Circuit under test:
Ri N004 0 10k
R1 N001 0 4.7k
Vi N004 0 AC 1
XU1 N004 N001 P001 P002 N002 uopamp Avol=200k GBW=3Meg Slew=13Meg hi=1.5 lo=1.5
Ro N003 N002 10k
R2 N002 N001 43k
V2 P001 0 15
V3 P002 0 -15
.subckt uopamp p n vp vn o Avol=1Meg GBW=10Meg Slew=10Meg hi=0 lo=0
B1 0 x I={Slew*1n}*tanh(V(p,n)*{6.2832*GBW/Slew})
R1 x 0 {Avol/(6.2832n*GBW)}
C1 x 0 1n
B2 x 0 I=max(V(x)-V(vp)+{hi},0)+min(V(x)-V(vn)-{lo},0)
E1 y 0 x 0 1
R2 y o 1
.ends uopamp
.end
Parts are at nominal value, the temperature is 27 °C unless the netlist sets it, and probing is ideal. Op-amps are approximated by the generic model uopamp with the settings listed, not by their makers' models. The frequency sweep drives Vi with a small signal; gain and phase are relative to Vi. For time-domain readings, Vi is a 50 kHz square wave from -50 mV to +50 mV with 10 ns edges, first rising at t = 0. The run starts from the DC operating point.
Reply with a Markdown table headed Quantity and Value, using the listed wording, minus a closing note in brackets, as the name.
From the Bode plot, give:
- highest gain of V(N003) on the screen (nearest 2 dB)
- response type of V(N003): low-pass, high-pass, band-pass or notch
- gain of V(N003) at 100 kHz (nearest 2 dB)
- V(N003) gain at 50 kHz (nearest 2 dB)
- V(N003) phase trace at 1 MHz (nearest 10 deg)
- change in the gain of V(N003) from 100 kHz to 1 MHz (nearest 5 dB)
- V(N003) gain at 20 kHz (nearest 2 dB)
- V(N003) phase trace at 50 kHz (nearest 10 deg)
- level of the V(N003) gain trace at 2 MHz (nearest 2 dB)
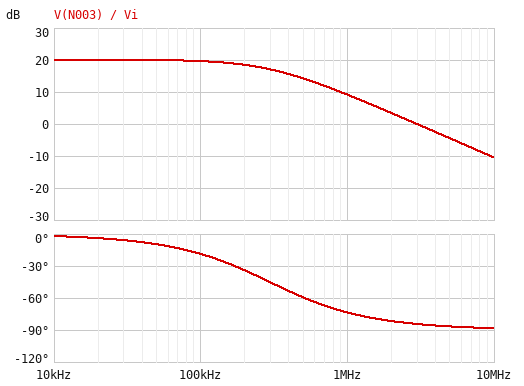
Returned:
| Quantity | Value |
|---|---|
| highest gain of V(N003) on the screen | 20 dB |
| response type of V(N003): low-pass, high-pass, band-pass or notch | low-pass |
| gain of V(N003) at 100 kHz | 20 dB |
| V(N003) gain at 50 kHz | 20 dB |
| V(N003) phase trace at 1 MHz | -70 deg |
| change in the gain of V(N003) from 100 kHz to 1 MHz | -10 dB |
| V(N003) gain at 20 kHz | 20 dB |
| V(N003) phase trace at 50 kHz | -10 deg |
| level of the V(N003) gain trace at 2 MHz | 4 dB |
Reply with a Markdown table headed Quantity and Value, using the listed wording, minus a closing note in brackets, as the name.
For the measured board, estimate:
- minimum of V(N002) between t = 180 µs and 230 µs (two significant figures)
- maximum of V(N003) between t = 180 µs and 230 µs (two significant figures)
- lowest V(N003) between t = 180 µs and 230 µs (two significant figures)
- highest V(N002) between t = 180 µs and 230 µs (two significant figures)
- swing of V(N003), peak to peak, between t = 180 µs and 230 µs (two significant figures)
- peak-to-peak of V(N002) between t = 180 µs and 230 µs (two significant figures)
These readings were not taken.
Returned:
| Quantity | Value |
|---|---|
| minimum of V(N002) between t = 180 µs and 230 µs | -510 mV |
| maximum of V(N003) between t = 180 µs and 230 µs | 510 mV |
| lowest V(N003) between t = 180 µs and 230 µs | -510 mV |
| highest V(N002) between t = 180 µs and 230 µs | 510 mV |
| swing of V(N003), peak to peak, between t = 180 µs and 230 µs | 1.0 V |
| peak-to-peak of V(N002) between t = 180 µs and 230 µs | 1.0 V |
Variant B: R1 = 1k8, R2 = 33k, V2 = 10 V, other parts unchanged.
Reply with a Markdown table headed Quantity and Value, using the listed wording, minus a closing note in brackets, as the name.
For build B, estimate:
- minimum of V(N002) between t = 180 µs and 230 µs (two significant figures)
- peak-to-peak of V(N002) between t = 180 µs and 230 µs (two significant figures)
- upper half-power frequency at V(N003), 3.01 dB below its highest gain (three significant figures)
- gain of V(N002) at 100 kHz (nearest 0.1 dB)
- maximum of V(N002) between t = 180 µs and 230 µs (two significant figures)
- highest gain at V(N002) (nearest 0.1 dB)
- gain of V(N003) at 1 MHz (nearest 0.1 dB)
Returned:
| Quantity | Value |
|---|---|
| minimum of V(N002) between t = 180 µs and 230 µs | -970 mV |
| peak-to-peak of V(N002) between t = 180 µs and 230 µs | 1.9 V |
| upper half-power frequency at V(N003), 3.01 dB below its highest gain | 155 kHz |
| gain of V(N002) at 100 kHz | 24.2 dB |
| maximum of V(N002) between t = 180 µs and 230 µs | 970 mV |
| highest gain at V(N002) | 25.7 dB |
| gain of V(N003) at 1 MHz | 9.4 dB |
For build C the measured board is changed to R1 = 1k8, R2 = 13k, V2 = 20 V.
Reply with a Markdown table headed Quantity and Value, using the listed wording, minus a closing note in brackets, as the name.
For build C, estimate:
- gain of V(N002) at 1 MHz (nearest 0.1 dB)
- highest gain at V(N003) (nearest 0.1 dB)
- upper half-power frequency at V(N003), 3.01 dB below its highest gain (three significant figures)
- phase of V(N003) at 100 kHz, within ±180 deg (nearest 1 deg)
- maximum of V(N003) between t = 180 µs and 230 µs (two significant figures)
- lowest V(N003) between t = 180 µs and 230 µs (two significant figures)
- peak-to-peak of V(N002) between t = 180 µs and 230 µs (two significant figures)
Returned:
| Quantity | Value |
|---|---|
| gain of V(N002) at 1 MHz | 9.0 dB |
| highest gain at V(N003) | 18.3 dB |
| upper half-power frequency at V(N003), 3.01 dB below its highest gain | 365 kHz |
| phase of V(N003) at 100 kHz, within ±180 deg | -15 deg |
| maximum of V(N003) between t = 180 µs and 230 µs | 410 mV |
| lowest V(N003) between t = 180 µs and 230 µs | -410 mV |
| peak-to-peak of V(N002) between t = 180 µs and 230 µs | 820 mV |
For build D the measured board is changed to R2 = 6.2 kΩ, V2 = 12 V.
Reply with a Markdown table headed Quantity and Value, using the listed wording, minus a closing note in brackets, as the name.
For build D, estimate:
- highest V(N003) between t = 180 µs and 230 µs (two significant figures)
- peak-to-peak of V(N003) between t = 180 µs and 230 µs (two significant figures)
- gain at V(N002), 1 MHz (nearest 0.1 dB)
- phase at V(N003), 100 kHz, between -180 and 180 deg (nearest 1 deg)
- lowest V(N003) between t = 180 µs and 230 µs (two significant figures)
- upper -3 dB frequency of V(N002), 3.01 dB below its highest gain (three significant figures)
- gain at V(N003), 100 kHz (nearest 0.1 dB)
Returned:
| Quantity | Value |
|---|---|
| highest V(N003) between t = 180 µs and 230 µs | 120 mV |
| peak-to-peak of V(N003) between t = 180 µs and 230 µs | 230 mV |
| gain at V(N002), 1 MHz | 5.3 dB |
| phase at V(N003), 100 kHz, between -180 and 180 deg | -4 deg |
| lowest V(N003) between t = 180 µs and 230 µs | -120 mV |
| upper -3 dB frequency of V(N002), 3.01 dB below its highest gain | 1.29 MHz |
| gain at V(N003), 100 kHz | 7.3 dB |
